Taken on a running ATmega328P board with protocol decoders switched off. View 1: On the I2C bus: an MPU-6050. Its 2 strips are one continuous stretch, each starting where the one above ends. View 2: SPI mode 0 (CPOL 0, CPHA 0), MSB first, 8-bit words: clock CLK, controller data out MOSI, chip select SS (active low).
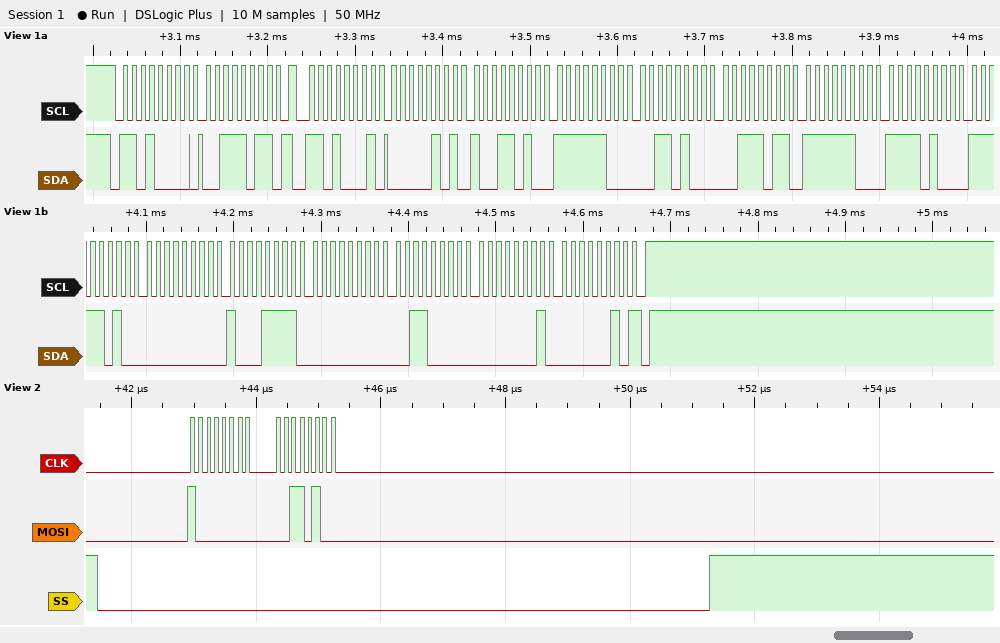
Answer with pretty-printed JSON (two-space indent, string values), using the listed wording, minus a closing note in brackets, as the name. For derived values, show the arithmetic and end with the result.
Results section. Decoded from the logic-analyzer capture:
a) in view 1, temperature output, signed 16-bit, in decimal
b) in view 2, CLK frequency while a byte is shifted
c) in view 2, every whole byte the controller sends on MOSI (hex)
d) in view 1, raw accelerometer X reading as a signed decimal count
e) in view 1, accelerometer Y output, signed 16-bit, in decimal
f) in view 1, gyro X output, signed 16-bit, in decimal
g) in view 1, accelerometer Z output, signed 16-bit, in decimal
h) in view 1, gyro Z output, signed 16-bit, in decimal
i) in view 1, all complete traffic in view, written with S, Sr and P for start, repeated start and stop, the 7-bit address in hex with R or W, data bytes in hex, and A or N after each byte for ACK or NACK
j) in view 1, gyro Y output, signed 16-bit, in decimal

{
  "in view 1, temperature output, signed 16-bit, in decimal": "0xF4FA = -2822",
  "in view 2, CLK frequency while a byte is shifted": "8 MHz",
  "in view 2, every whole byte the controller sends on MOSI": "80 34",
  "in view 1, raw accelerometer X reading as a signed decimal count": "0x059A = 1434",
  "in view 1, accelerometer Y output, signed 16-bit, in decimal": "0xFC34 = -972",
  "in view 1, gyro X output, signed 16-bit, in decimal": "0x008F = 143",
  "in view 1, accelerometer Z output, signed 16-bit, in decimal": "0x3BFC = 15356",
  "in view 1, gyro Z output, signed 16-bit, in decimal": "0x0102 = 258",
  "in view 1, all complete traffic in view, written with S, Sr and P for start, repeated start and stop, the 7-bit address in hex with R or W, data bytes in hex, and A or N after each byte for ACK or NACK": "S 68W A 3B A Sr 68R A 05 A 9A A FC A 34 A 3B A FC A F4 A FA A 00 A 8F A 00 A 30 A 01 A 02 N P",
  "in view 1, gyro Y output, signed 16-bit, in decimal": "0x0030 = 48"
}
